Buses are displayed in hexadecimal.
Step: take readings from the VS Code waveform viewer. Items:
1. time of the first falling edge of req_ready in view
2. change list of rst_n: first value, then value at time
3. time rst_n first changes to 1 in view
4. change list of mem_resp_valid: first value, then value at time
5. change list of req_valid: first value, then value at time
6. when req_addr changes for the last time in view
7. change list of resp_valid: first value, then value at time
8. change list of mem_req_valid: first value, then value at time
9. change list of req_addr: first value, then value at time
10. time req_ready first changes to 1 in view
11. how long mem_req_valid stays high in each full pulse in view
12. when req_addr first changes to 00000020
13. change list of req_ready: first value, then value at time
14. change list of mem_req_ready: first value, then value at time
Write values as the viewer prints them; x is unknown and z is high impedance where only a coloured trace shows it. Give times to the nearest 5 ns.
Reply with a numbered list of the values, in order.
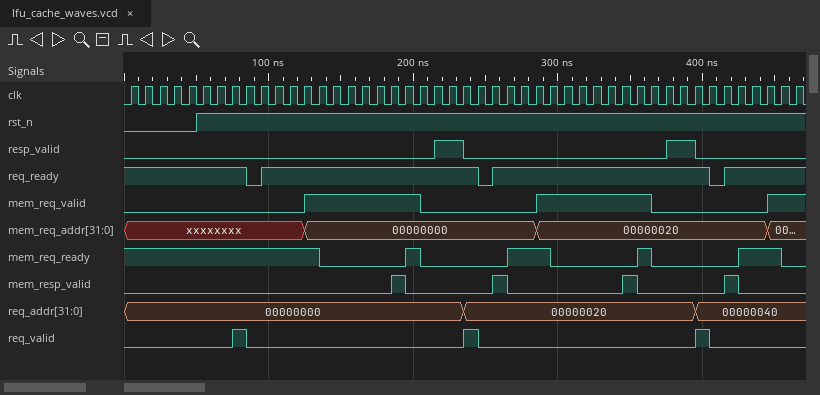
1. 85 ns
2. 0, 1 at 50 ns
3. 50 ns
4. 0, 1 at 185 ns, 0 at 195 ns, 1 at 255 ns, 0 at 265 ns, 1 at 345 ns, 0 at 355 ns, 1 at 415 ns, 0 at 425 ns
5. 0, 1 at 75 ns, 0 at 85 ns, 1 at 235 ns, 0 at 245 ns, 1 at 395 ns, 0 at 405 ns
6. 395 ns
7. 0, 1 at 215 ns, 0 at 235 ns, 1 at 375 ns, 0 at 395 ns
8. 0, 1 at 125 ns, 0 at 205 ns, 1 at 285 ns, 0 at 365 ns, 1 at 445 ns
9. 00000000, 00000020 at 235 ns, 00000040 at 395 ns
10. 95 ns
11. 80 ns, 80 ns
12. 235 ns
13. 1, 0 at 85 ns, 1 at 95 ns, 0 at 245 ns, 1 at 255 ns, 0 at 405 ns, 1 at 415 ns
14. 1, 0 at 135 ns, 1 at 195 ns, 0 at 205 ns, 1 at 265 ns, 0 at 295 ns, 1 at 355 ns, 0 at 365 ns, 1 at 425 ns, 0 at 455 ns
